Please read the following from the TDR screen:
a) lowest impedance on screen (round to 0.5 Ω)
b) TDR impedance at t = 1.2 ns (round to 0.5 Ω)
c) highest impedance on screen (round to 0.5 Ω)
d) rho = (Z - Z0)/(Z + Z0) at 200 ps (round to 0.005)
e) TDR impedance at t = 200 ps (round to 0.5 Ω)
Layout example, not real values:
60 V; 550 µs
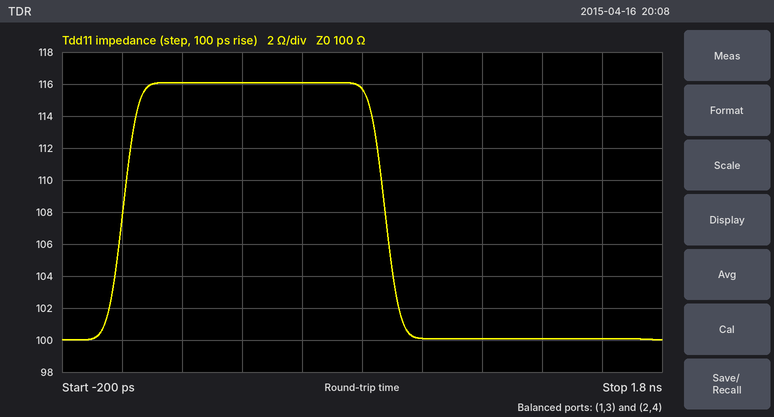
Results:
100.0 Ω; 100.0 Ω; 116.0 Ω; +0.075; 116.0 Ω
